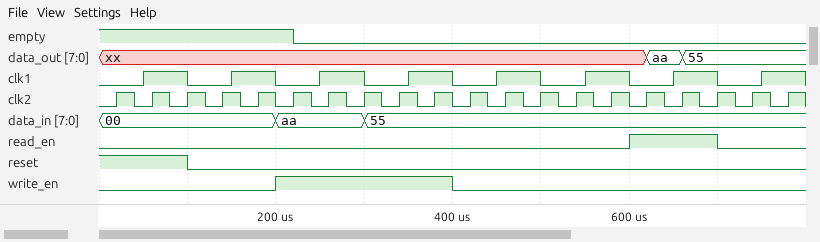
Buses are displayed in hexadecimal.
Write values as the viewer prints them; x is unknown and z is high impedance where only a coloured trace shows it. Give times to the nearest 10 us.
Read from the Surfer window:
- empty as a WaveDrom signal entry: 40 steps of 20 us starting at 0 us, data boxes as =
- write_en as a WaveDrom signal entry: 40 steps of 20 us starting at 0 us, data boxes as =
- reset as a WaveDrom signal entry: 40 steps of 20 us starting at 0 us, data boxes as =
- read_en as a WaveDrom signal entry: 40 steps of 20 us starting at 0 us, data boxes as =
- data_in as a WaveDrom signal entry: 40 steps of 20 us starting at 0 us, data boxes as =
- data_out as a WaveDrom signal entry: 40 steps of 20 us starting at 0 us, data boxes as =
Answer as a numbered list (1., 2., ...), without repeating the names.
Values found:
1. {name: 'empty', wave: '1..........0............................'}
2. {name: 'write_en', wave: '0.........1.........0...................'}
3. {name: 'reset', wave: '1....0..................................'}
4. {name: 'read_en', wave: '0.............................1....0....'}
5. {name: 'data_in', wave: '=.........=....=........................', data: '00 aa 55'}
6. {name: 'data_out', wave: 'x..............................=.=......', data: 'aa 55'}
